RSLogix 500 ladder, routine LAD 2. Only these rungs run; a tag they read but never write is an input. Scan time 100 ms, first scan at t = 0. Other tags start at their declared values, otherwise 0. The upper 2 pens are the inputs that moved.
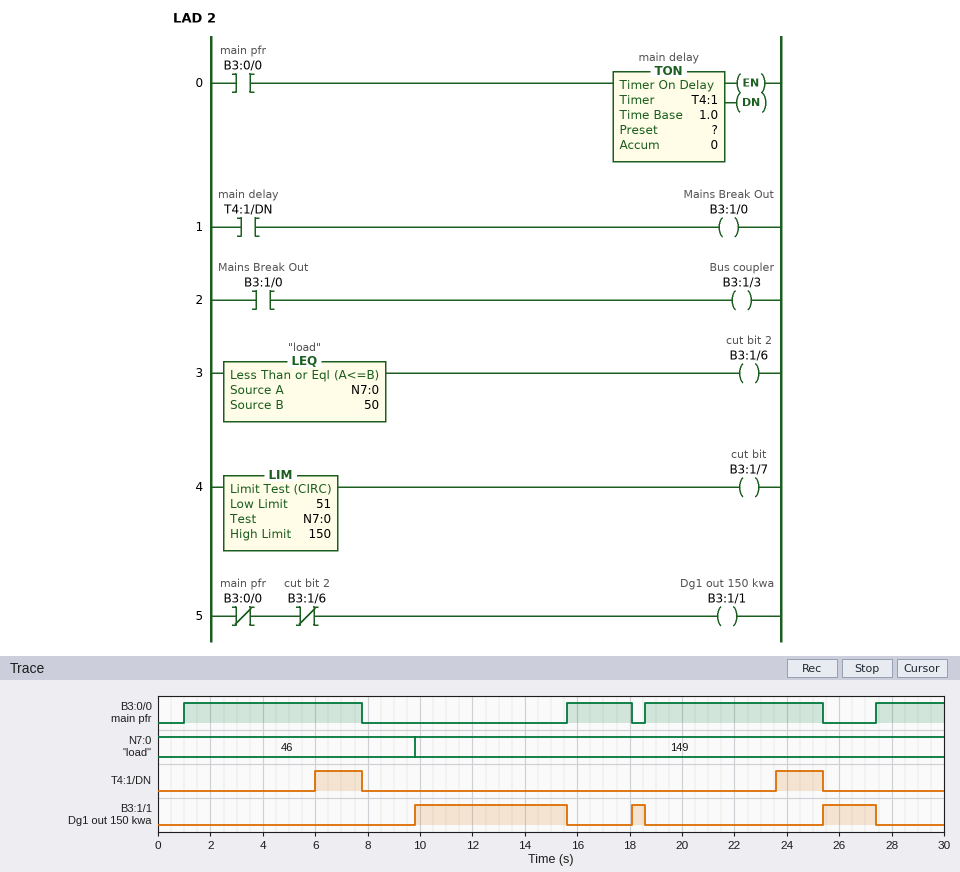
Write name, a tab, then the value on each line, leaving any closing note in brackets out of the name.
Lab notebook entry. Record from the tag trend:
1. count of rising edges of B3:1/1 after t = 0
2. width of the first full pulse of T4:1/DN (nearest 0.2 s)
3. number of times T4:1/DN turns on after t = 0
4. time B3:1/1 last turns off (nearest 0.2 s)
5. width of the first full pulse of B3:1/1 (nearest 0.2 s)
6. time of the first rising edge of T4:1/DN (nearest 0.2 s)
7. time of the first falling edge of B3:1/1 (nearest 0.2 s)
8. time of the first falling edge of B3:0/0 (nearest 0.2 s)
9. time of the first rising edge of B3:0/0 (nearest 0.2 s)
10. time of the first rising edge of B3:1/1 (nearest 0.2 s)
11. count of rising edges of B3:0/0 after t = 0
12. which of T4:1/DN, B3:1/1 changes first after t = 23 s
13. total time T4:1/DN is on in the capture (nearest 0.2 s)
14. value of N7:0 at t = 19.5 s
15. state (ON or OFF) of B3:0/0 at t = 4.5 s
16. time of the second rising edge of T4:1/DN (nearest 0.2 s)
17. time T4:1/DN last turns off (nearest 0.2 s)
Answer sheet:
count of rising edges of B3:1/1 after t = 0	3
width of the first full pulse of T4:1/DN	1.8 s
number of times T4:1/DN turns on after t = 0	2
time B3:1/1 last turns off	27.4 s
width of the first full pulse of B3:1/1	5.8 s
time of the first rising edge of T4:1/DN	6.0 s
time of the first falling edge of B3:1/1	15.6 s
time of the first falling edge of B3:0/0	7.8 s
time of the first rising edge of B3:0/0	1.0 s
time of the first rising edge of B3:1/1	9.8 s
count of rising edges of B3:0/0 after t = 0	4
which of T4:1/DN, B3:1/1 changes first after t = 23 s	T4:1/DN
total time T4:1/DN is on in the capture	3.6 s
value of N7:0 at t = 19.5 s	149
state (ON or OFF) of B3:0/0 at t = 4.5 s	ON
time of the second rising edge of T4:1/DN	23.6 s
time T4:1/DN last turns off	25.4 s
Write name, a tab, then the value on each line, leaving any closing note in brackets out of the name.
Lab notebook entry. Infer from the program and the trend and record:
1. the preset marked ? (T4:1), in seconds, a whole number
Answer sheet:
the preset marked ? (T4:1), in seconds, a whole number	5 s
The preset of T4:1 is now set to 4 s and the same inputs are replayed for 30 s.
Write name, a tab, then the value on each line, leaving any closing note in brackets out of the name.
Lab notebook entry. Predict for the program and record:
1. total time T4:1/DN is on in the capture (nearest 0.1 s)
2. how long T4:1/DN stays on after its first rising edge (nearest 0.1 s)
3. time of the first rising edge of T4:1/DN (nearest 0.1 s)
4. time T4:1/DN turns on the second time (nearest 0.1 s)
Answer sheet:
total time T4:1/DN is on in the capture	5.6 s
how long T4:1/DN stays on after its first rising edge	2.8 s
time of the first rising edge of T4:1/DN	5.0 s
time T4:1/DN turns on the second time	22.6 s
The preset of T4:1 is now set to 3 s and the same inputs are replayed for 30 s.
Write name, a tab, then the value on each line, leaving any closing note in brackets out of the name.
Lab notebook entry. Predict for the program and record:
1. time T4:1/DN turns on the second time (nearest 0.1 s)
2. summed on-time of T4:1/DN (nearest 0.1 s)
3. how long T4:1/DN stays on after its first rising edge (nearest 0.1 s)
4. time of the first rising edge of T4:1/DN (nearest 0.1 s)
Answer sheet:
time T4:1/DN turns on the second time	21.6 s
summed on-time of T4:1/DN	7.6 s
how long T4:1/DN stays on after its first rising edge	3.8 s
time of the first rising edge of T4:1/DN	4.0 s
